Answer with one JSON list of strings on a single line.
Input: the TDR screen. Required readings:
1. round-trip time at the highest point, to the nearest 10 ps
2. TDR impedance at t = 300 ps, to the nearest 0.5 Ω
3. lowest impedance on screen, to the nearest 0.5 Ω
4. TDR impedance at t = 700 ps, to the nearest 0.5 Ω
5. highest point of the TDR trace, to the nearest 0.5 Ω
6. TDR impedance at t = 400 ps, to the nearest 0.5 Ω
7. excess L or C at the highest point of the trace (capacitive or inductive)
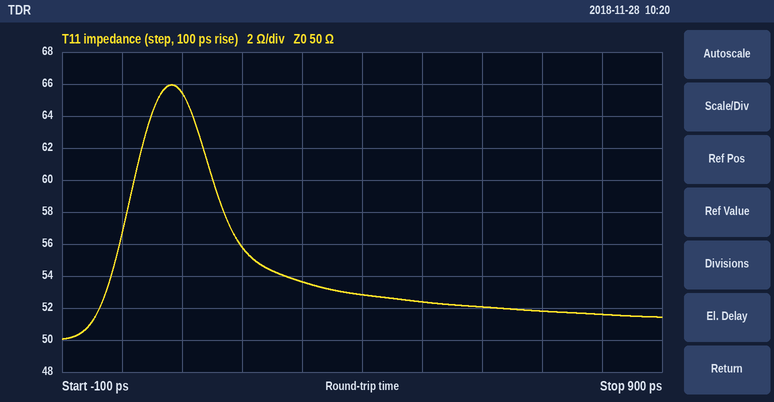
["80 ps", "53.5 Ω", "50.0 Ω", "52.0 Ω", "66.0 Ω", "53.0 Ω", "inductive"]
